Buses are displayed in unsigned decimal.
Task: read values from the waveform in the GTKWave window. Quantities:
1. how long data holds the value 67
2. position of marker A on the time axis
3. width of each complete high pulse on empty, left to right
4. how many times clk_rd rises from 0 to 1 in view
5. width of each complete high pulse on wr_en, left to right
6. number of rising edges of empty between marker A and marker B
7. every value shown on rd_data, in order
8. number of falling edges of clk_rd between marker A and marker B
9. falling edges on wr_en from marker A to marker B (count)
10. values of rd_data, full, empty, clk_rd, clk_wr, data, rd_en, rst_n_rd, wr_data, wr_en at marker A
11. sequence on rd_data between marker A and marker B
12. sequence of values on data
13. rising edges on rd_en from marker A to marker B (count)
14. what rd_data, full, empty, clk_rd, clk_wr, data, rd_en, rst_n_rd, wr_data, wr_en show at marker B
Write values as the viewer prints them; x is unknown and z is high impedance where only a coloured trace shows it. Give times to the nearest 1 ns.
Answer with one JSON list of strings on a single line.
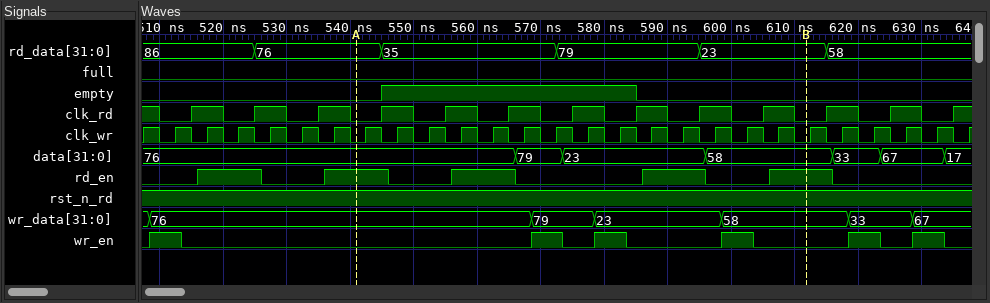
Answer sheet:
["10 ns", "541 ns", "40 ns", "13", "5 ns, 5 ns, 5 ns, 5 ns, 5 ns, 5 ns", "1", "86, 76, 35, 79, 23, 58", "7", "3", "rd_data=76, full=0, empty=0, clk_rd=0, clk_wr=0, data=76, rd_en=1, rst_n_rd=1, wr_data=76, wr_en=0", "76, 35, 79, 23", "76, 79, 23, 58, 33, 67, 17", "3", "rd_data=23, full=0, empty=0, clk_rd=0, clk_wr=0, data=58, rd_en=1, rst_n_rd=1, wr_data=58, wr_en=0"]
